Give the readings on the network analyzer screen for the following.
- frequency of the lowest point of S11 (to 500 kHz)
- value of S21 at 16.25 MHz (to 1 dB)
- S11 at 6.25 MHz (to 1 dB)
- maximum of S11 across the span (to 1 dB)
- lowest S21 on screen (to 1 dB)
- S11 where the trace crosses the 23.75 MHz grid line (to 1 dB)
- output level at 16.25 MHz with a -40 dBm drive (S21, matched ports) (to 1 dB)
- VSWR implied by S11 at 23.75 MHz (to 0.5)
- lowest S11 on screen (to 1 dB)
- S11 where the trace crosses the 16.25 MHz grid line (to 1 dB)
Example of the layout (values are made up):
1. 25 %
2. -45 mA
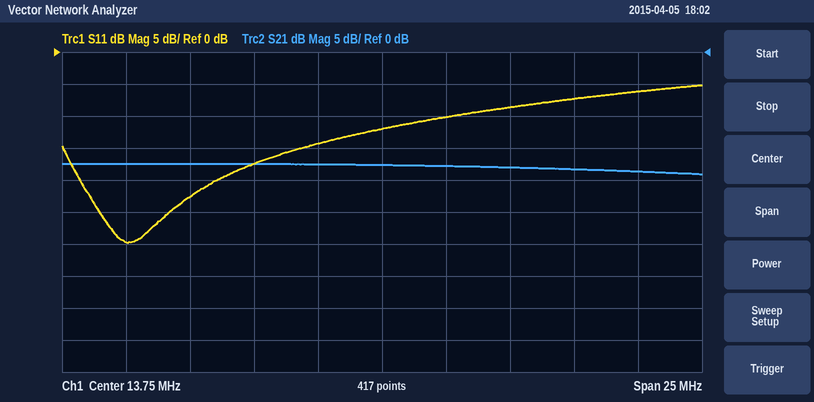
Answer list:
1. 4.0 MHz
2. -18 dB
3. -23 dB
4. -5 dB
5. -19 dB
6. -6 dB
7. -58 dBm
8. 3.0
9. -30 dB
10. -10 dB
